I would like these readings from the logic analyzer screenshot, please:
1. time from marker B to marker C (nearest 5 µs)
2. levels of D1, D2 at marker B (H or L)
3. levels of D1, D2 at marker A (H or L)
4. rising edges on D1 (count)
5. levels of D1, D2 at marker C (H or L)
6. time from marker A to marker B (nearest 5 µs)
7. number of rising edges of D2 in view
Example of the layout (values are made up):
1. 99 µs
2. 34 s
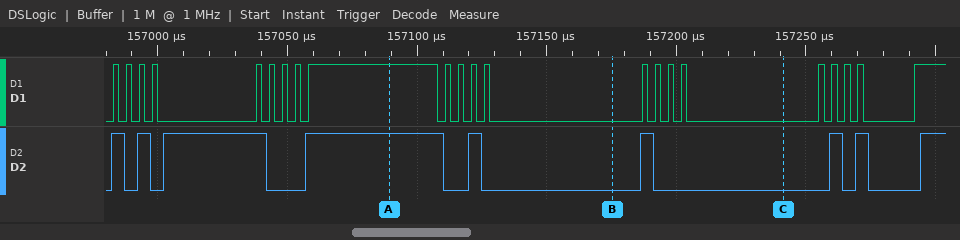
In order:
1. 65 µs
2. D1=L, D2=L
3. D1=H, D2=H
4. 22
5. D1=L, D2=L
6. 85 µs
7. 9
